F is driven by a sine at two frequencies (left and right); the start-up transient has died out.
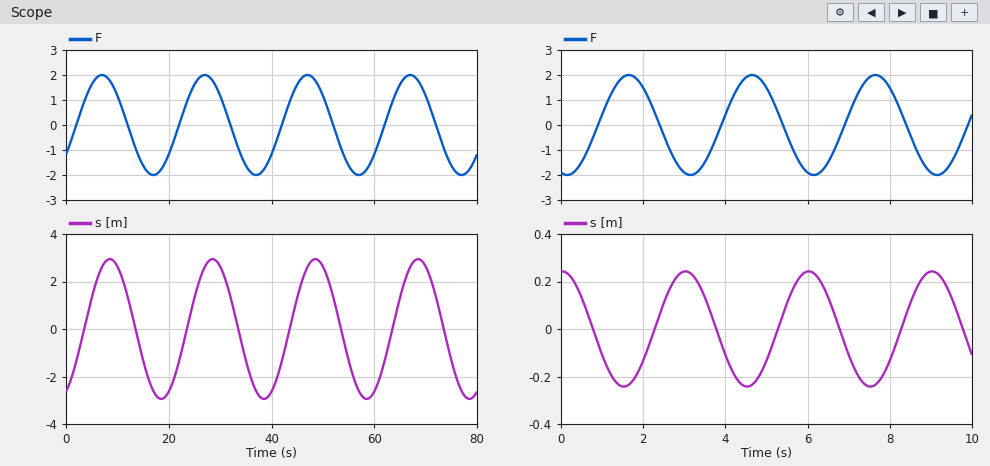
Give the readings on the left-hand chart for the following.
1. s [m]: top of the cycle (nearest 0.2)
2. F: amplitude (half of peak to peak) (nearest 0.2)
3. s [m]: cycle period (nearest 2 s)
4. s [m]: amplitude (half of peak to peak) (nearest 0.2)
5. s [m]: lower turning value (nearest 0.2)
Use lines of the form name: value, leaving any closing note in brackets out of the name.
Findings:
s [m]: top of the cycle: 3.0
F: amplitude (half of peak to peak): 2.0
s [m]: cycle period: 20 s
s [m]: amplitude (half of peak to peak): 3.0
s [m]: lower turning value: -3.0
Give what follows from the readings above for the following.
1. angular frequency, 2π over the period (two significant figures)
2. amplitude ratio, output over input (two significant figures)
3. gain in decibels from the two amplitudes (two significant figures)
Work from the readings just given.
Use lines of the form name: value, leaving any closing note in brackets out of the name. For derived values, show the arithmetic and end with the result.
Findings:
angular frequency, 2π over the period: 2π / 20 = 0.31 rad/s
amplitude ratio, output over input: 3 / 2 = 1.5
gain in decibels from the two amplitudes: 20 log10(3 / 2) = 3.5 dB
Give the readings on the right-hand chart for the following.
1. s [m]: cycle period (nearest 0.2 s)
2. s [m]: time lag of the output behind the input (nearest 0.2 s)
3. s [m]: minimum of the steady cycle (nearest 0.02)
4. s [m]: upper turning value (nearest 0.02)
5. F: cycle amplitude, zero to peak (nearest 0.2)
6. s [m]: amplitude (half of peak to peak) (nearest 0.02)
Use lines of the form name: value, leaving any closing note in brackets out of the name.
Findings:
s [m]: cycle period: 3.0 s
s [m]: time lag of the output behind the input: 1.4 s
s [m]: minimum of the steady cycle: -0.24
s [m]: upper turning value: 0.24
F: cycle amplitude, zero to peak: 2.0
s [m]: amplitude (half of peak to peak): 0.24
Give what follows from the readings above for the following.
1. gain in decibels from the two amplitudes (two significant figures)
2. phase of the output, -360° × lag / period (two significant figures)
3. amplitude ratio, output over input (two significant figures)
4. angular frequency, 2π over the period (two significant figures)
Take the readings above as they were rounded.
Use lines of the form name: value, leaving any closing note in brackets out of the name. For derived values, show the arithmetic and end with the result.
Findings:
gain in decibels from the two amplitudes: 20 log10(0.24 / 2) = -18 dB
phase of the output, -360° × lag / period: -360 × 1.4 / 3 = -170°
amplitude ratio, output over input: 0.24 / 2 = 0.12
angular frequency, 2π over the period: 2π / 3 = 2.1 rad/s
